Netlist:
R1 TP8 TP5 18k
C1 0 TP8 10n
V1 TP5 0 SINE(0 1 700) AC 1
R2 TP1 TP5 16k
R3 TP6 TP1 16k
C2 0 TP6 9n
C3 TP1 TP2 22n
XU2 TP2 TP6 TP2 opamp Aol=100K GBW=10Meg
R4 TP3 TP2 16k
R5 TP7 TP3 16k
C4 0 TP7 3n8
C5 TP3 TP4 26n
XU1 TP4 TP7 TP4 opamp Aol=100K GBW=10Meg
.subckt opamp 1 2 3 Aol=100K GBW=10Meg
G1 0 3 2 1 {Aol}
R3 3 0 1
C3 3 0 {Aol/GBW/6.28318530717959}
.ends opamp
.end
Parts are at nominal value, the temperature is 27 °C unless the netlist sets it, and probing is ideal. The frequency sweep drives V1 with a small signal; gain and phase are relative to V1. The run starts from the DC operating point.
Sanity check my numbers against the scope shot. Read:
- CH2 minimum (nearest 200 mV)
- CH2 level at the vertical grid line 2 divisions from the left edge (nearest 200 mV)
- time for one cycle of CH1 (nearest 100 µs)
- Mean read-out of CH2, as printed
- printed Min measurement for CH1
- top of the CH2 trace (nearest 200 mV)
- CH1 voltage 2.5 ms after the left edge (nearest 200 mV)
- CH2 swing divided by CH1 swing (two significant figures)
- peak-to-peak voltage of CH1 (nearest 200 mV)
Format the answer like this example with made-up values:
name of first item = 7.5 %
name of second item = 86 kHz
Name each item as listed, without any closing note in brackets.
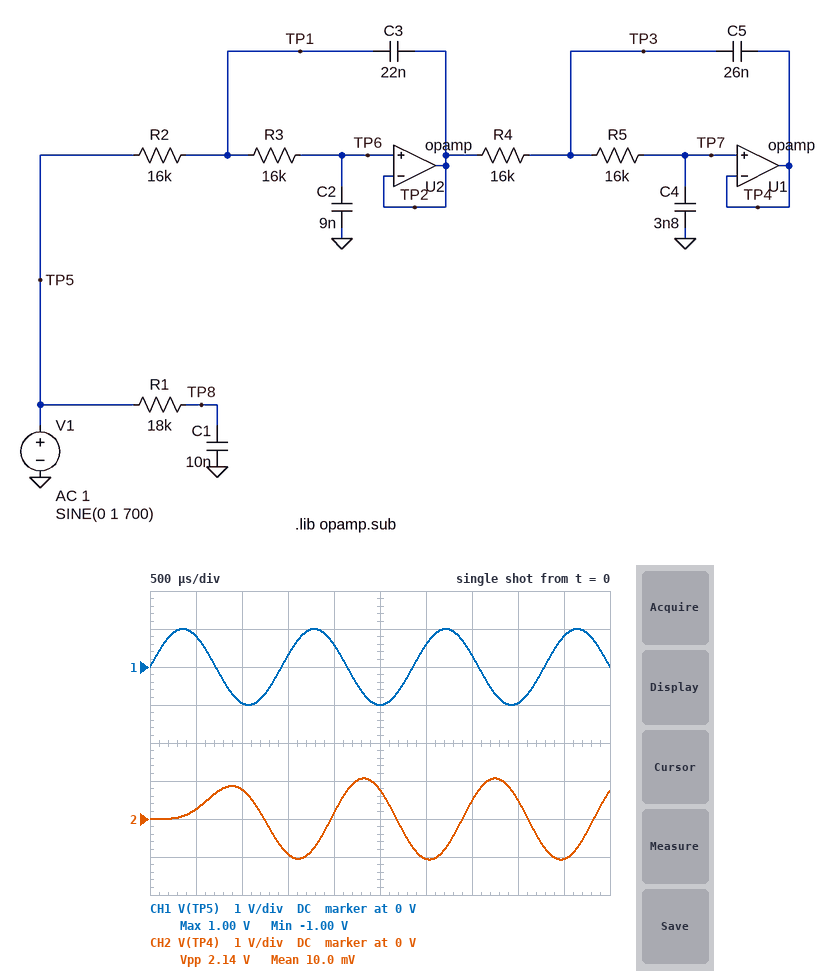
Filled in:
CH2 minimum = -1.0 V
CH2 level at the vertical grid line 2 divisions from the left edge = 800 mV
time for one cycle of CH1 = 1.4 ms
Mean read-out of CH2, as printed = 10.0 mV
printed Min measurement for CH1 = -1.00 V
top of the CH2 trace = 1.0 V
CH1 voltage 2.5 ms after the left edge = -1.0 V
CH2 swing divided by CH1 swing = 1.1
peak-to-peak voltage of CH1 = 2.0 V
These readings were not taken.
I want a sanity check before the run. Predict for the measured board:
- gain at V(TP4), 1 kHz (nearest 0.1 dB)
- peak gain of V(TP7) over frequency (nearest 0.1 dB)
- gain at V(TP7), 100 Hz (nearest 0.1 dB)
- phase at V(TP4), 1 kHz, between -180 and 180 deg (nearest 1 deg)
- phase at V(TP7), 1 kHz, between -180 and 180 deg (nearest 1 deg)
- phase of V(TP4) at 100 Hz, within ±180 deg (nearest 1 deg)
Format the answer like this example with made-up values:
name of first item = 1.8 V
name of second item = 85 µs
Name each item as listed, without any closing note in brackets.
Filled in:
gain at V(TP4), 1 kHz = -4.0 dB
peak gain of V(TP7) over frequency = 1.2 dB
gain at V(TP7), 100 Hz = 0.1 dB
phase at V(TP4), 1 kHz, between -180 and 180 deg = 151 deg
phase at V(TP7), 1 kHz, between -180 and 180 deg = 151 deg
phase of V(TP4) at 100 Hz, within ±180 deg = -15 deg
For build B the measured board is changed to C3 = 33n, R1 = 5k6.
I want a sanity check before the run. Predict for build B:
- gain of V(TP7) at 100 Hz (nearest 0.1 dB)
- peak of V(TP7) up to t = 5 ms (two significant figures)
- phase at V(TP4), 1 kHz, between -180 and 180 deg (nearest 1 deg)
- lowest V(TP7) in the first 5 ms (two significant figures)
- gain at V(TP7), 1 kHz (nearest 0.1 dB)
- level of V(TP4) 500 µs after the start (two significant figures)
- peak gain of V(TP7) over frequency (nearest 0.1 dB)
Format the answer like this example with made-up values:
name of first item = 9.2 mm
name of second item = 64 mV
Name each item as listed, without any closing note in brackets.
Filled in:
gain of V(TP7) at 100 Hz = 0.2 dB
peak of V(TP7) up to t = 5 ms = 1.0 V
phase at V(TP4), 1 kHz, between -180 and 180 deg = 132 deg
lowest V(TP7) in the first 5 ms = -1.0 V
gain at V(TP7), 1 kHz = -6.3 dB
level of V(TP4) 500 µs after the start = 200 mV
peak gain of V(TP7) over frequency = 2.1 dB
